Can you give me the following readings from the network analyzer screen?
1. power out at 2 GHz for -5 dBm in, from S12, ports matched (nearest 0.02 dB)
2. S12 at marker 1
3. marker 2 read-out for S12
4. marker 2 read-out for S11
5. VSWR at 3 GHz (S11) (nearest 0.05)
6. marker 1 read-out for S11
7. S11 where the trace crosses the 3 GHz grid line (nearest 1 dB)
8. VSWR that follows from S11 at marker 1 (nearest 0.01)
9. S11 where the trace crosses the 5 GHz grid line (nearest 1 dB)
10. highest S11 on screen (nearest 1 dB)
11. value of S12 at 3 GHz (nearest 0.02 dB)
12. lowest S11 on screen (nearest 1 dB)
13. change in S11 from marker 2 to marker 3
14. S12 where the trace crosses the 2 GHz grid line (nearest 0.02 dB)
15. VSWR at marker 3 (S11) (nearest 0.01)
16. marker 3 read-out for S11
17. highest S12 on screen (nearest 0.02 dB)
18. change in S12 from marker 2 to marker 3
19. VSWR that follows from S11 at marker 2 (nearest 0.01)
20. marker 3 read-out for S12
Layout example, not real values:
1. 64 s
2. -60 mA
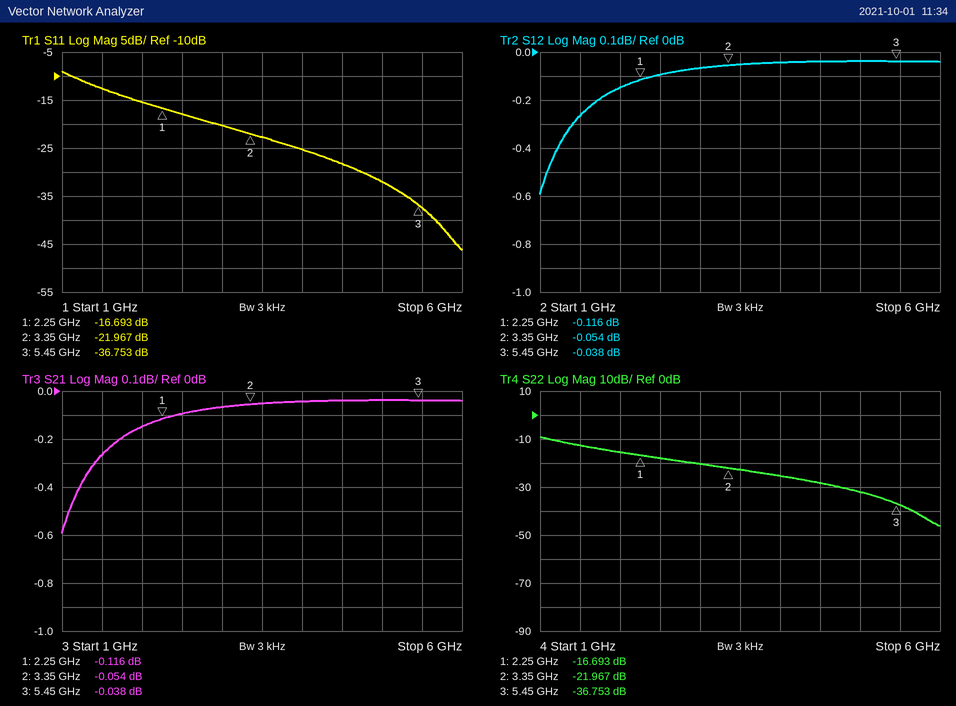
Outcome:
1. -5.14 dBm
2. -0.116 dB
3. -0.054 dB
4. -21.967 dB
5. 1.20
6. -16.693 dB
7. -20 dB
8. 1.34
9. -32 dB
10. -9 dB
11. -0.06 dB
12. -46 dB
13. -14.786 dB
14. -0.14 dB
15. 1.03
16. -36.753 dB
17. -0.04 dB
18. 0.016 dB
19. 1.17
20. -0.038 dB
